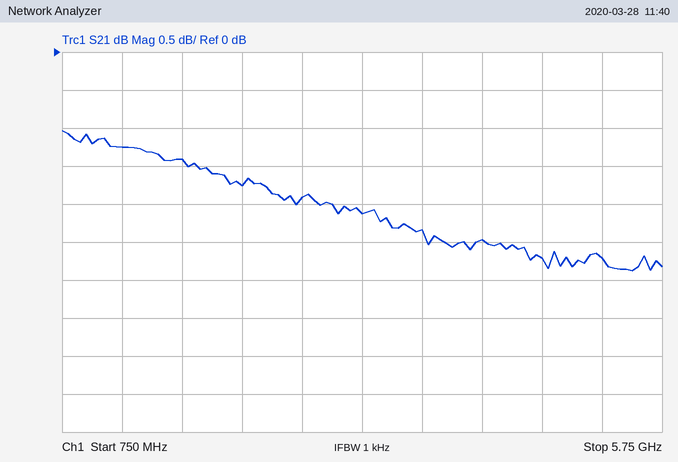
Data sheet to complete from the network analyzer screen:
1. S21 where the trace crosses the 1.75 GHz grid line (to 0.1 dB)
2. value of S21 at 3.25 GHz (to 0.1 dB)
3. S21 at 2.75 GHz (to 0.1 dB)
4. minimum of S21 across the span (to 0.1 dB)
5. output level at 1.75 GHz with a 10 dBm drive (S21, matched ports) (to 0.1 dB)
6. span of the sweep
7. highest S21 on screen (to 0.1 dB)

-1.4 dB
-2.1 dB
-1.9 dB
-2.9 dB
8.6 dBm
5 GHz
-1.0 dB
